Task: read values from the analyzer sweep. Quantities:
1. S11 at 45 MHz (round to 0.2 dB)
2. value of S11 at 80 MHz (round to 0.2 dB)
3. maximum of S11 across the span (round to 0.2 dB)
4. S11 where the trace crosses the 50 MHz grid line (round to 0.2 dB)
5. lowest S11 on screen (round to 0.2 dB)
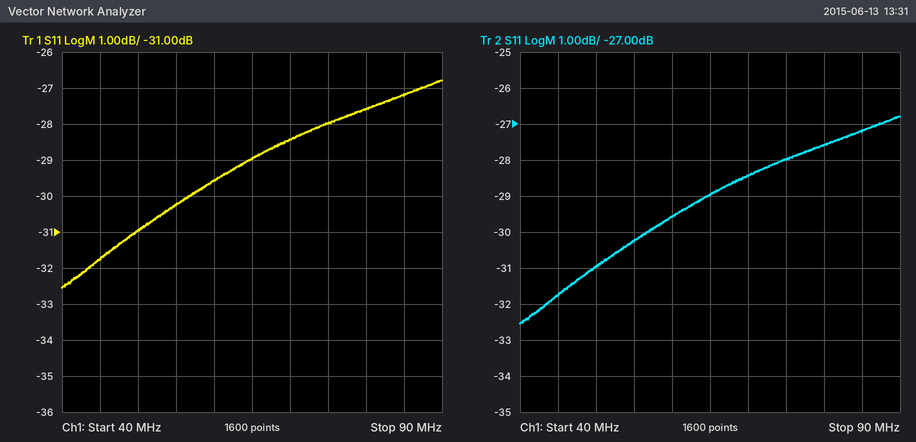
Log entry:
-31.8 dB
-27.6 dB
-26.8 dB
-31.0 dB
-32.6 dB
